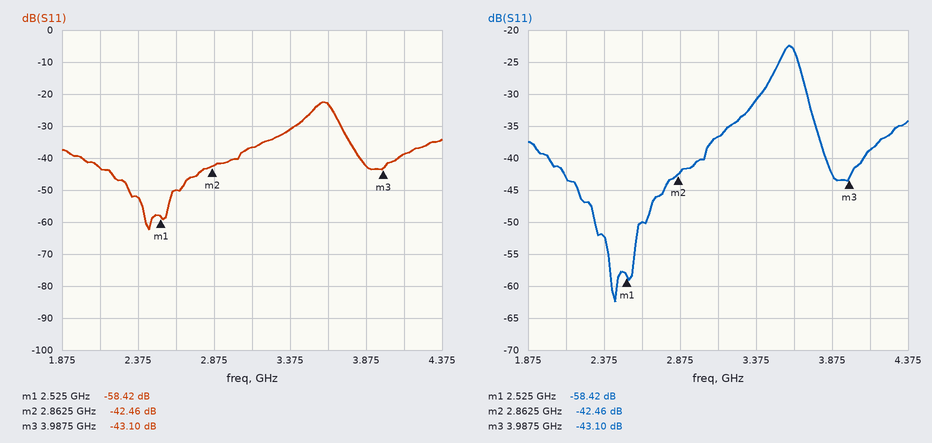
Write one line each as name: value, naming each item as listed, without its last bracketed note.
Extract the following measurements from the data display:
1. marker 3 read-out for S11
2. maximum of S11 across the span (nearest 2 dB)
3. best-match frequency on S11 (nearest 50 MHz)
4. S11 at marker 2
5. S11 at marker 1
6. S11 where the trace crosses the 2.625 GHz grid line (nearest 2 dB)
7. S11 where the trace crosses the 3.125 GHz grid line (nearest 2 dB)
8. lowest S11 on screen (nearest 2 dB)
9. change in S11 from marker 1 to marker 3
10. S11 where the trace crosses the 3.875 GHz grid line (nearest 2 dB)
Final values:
marker 3 read-out for S11: -43.10 dB
maximum of S11 across the span: -22 dB
best-match frequency on S11: 2.45 GHz
S11 at marker 2: -42.46 dB
S11 at marker 1: -58.42 dB
S11 where the trace crosses the 2.625 GHz grid line: -50 dB
S11 where the trace crosses the 3.125 GHz grid line: -36 dB
lowest S11 on screen: -62 dB
change in S11 from marker 1 to marker 3: 15.32 dB
S11 where the trace crosses the 3.875 GHz grid line: -42 dB
